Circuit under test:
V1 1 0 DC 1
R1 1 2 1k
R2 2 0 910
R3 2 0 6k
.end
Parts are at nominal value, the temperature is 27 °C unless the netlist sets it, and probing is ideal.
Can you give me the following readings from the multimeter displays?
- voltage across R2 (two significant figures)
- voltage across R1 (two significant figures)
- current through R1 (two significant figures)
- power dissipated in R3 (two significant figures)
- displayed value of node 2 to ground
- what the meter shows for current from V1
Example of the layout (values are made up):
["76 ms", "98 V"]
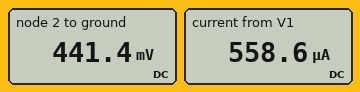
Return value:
["440 mV", "560 mV", "560 µA", "32 µW", "441.4 mV", "558.6 µA"]
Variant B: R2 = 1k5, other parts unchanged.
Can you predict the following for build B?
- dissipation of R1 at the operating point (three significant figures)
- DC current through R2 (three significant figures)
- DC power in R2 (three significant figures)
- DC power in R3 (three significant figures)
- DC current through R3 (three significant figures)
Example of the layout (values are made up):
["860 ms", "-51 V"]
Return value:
["207 µW", "364 µA", "198 µW", "49.6 µW", "90.9 µA"]
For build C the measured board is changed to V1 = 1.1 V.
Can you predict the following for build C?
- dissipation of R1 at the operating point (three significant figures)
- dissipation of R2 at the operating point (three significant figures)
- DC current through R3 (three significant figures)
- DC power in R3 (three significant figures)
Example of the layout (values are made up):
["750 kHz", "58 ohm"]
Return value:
["378 µW", "259 µW", "80.9 µA", "39.3 µW"]
